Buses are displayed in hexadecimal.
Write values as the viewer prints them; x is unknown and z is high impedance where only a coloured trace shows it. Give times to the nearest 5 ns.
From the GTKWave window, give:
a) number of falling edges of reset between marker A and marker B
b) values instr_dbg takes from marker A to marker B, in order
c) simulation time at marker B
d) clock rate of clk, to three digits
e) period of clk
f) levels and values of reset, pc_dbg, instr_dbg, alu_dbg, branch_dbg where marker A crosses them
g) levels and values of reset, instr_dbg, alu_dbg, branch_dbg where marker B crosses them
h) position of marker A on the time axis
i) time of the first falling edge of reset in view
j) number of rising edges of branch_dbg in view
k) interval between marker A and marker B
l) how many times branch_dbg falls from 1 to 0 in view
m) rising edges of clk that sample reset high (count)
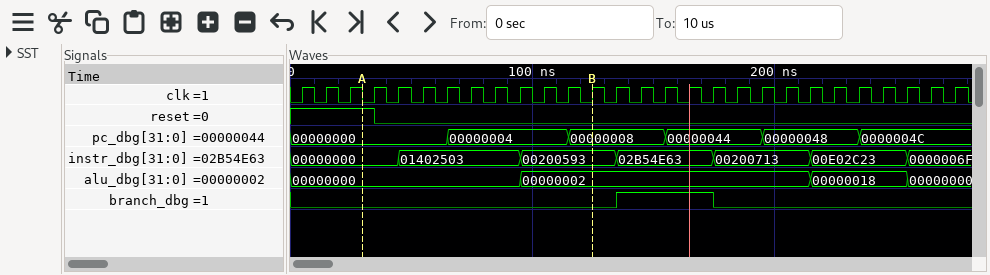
1
00000000, 01402503, 00200593
125 ns
100 MHz
10 ns
reset=1, pc_dbg=00000000, instr_dbg=00000000, alu_dbg=00000000, branch_dbg=0
reset=0, instr_dbg=00200593, alu_dbg=00000002, branch_dbg=0
30 ns
35 ns
1
95 ns
1
4
